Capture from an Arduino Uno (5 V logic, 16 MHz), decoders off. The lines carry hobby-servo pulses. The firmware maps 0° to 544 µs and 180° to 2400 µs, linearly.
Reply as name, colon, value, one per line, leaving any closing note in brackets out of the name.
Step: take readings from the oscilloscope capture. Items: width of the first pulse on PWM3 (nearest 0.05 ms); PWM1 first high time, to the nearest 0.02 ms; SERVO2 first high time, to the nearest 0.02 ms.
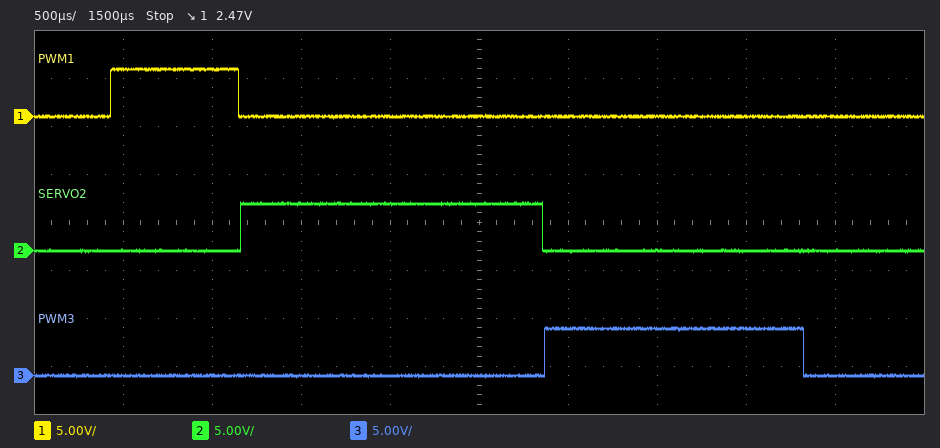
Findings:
width of the first pulse on PWM3: 1.45 ms
PWM1 first high time, to the nearest 0.02 ms: 0.72 ms
SERVO2 first high time, to the nearest 0.02 ms: 1.70 ms
